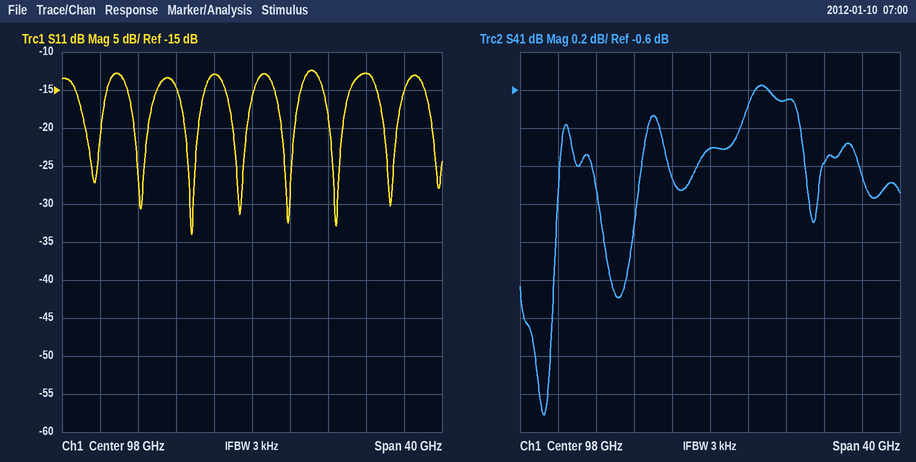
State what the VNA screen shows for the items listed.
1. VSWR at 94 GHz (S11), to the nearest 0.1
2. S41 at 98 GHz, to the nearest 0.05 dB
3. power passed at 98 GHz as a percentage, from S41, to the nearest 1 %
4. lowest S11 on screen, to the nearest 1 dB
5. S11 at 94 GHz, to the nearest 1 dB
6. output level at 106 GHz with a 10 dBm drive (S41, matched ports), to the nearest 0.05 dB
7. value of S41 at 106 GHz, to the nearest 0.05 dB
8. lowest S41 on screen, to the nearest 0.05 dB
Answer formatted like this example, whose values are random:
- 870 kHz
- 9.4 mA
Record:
- 1.6
- -0.90 dB
- 81 %
- -34 dB
- -13 dB
- 9.35 dBm
- -0.65 dB
- -2.30 dB
